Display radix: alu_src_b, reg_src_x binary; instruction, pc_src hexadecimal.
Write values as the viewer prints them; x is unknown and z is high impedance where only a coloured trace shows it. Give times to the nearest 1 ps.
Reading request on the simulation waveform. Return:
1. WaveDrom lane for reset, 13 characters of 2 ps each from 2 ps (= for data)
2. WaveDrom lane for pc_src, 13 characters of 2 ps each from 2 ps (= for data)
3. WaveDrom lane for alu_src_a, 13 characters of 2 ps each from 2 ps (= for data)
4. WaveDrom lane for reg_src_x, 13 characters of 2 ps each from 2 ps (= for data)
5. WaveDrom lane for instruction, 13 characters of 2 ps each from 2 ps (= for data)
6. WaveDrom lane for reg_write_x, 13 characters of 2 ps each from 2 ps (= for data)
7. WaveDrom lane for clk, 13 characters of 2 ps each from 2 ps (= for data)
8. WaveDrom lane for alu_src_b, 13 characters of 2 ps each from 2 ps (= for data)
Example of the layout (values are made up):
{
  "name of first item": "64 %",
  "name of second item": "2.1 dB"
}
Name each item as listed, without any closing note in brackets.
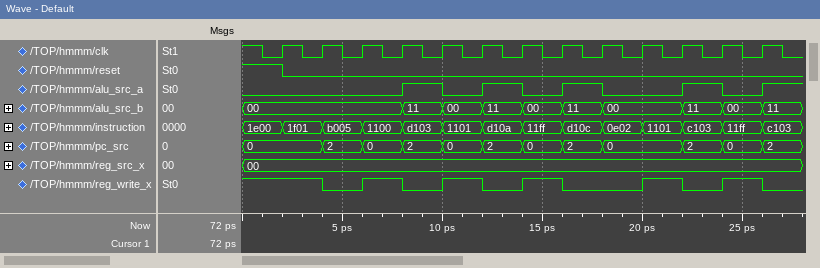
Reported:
{
  "WaveDrom lane for reset, 13 characters of 2 ps each from 2 ps": "{name: 'reset', wave: '0............'}",
  "WaveDrom lane for pc_src, 13 characters of 2 ps each from 2 ps": "{name: 'pc_src', wave: '=========.===', data: '0 2 0 2 0 2 0 2 0 2 0 2'}",
  "WaveDrom lane for alu_src_a, 13 characters of 2 ps each from 2 ps": "{name: 'alu_src_a', wave: '0..101010.101'}",
  "WaveDrom lane for reg_src_x, 13 characters of 2 ps each from 2 ps": "{name: 'reg_src_x', wave: '=............', data: '00'}",
  "WaveDrom lane for instruction, 13 characters of 2 ps each from 2 ps": "{name: 'instruction', wave: '=============', data: '1f01 b005 1100 d103 1101 d10a 11ff d10c 0e02 1101 c103 11ff c103'}",
  "WaveDrom lane for reg_write_x, 13 characters of 2 ps each from 2 ps": "{name: 'reg_write_x', wave: '10101010.1010'}",
  "WaveDrom lane for clk, 13 characters of 2 ps each from 2 ps": "{name: 'clk', wave: 'p............'}",
  "WaveDrom lane for alu_src_b, 13 characters of 2 ps each from 2 ps": "{name: 'alu_src_b', wave: '=..======.===', data: '00 11 00 11 00 11 00 11 00 11'}"
}
